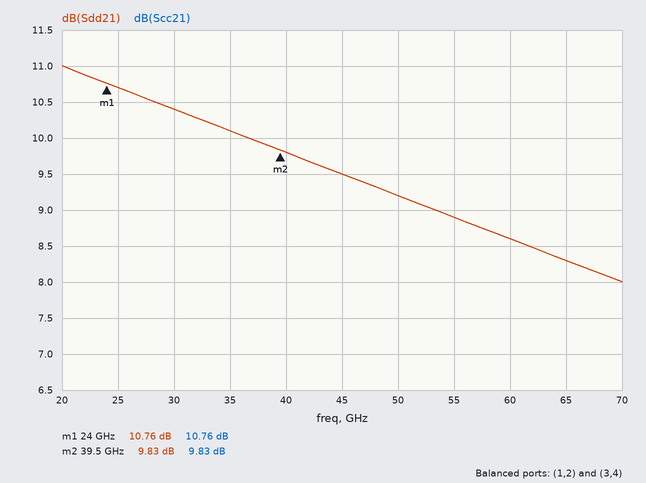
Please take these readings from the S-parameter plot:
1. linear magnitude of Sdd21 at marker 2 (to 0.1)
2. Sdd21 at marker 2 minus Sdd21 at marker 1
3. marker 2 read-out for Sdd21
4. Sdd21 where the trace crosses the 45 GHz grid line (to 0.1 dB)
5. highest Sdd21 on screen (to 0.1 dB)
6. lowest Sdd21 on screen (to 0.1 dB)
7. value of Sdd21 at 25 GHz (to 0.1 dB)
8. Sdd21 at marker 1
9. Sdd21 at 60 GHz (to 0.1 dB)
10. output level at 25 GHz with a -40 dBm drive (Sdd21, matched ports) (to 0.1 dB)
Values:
3.1
-0.93 dB
9.83 dB
9.5 dB
11.0 dB
8.0 dB
10.7 dB
10.76 dB
8.6 dB
-29.3 dBm
